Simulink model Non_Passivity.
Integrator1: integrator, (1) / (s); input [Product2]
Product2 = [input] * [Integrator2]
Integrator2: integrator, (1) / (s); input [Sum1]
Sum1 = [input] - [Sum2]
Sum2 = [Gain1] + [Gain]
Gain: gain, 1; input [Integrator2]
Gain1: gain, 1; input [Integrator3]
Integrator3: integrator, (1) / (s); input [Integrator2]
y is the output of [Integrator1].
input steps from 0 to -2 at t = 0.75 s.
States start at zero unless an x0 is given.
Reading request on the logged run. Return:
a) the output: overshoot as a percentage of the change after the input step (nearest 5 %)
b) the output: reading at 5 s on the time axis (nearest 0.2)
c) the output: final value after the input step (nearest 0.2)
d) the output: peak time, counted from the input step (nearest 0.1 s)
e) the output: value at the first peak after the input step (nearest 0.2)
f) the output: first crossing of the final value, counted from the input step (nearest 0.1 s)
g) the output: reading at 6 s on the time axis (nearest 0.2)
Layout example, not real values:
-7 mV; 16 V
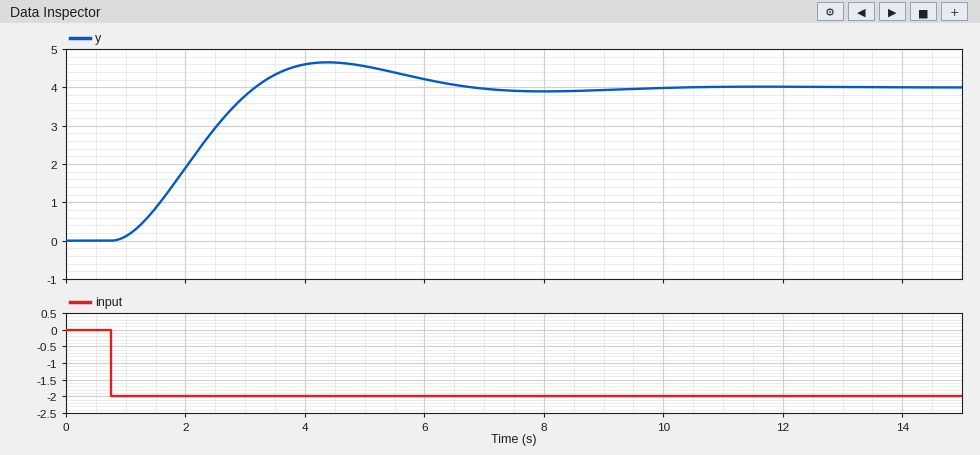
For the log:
15 %; 4.6; 4.0; 3.6 s; 4.6; 2.4 s; 4.2
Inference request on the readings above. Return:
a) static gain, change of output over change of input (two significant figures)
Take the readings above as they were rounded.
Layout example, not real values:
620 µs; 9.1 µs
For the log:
-2.0
